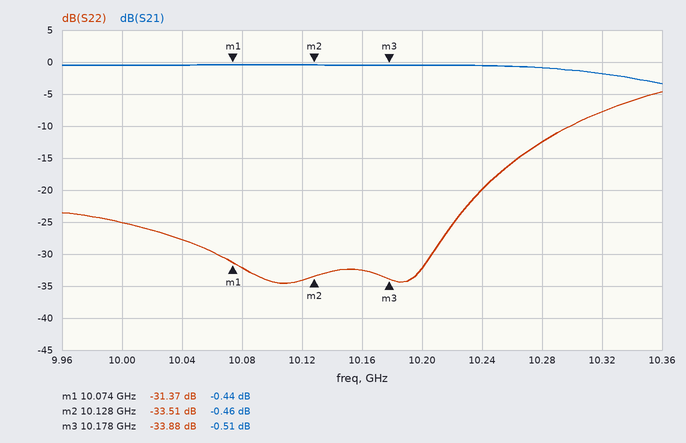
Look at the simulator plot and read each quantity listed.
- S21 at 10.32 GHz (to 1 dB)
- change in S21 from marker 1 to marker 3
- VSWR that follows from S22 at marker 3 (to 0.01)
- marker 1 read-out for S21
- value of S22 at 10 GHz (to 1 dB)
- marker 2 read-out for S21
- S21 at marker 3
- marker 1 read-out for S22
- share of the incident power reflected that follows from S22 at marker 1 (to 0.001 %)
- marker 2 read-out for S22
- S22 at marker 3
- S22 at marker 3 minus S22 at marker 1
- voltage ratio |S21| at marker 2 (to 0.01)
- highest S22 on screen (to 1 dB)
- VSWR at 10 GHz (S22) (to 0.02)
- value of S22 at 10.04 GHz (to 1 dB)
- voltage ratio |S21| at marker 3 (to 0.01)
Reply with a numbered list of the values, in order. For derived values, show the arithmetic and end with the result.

1. -2 dB
2. -0.51 − (-0.44) = -0.07 dB
3. (1 + 0.0202)/(1 − 0.0202) ≈ 1.04
4. -0.44 dB
5. -25 dB
6. -0.46 dB
7. -0.51 dB
8. -31.37 dB
9. 10^(-31.37/10) ≈ 0.073 %
10. -33.51 dB
11. -33.88 dB
12. -33.88 − (-31.37) = -2.51 dB
13. 10^(-0.46/20) ≈ 0.95
14. -5 dB
15. |Γ| = 10^(-25/20) = 0.0562; VSWR = (1 + 0.0562)/(1 − 0.0562) ≈ 1.12
16. -28 dB
17. 10^(-0.51/20) ≈ 0.94
